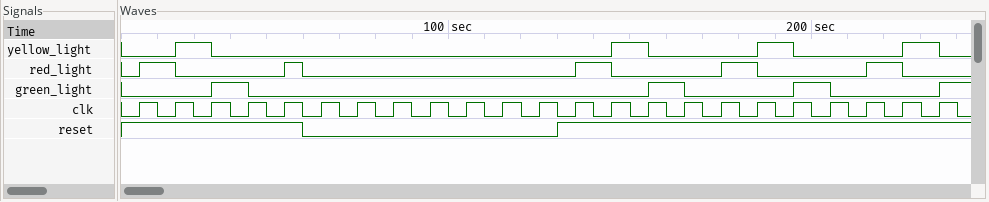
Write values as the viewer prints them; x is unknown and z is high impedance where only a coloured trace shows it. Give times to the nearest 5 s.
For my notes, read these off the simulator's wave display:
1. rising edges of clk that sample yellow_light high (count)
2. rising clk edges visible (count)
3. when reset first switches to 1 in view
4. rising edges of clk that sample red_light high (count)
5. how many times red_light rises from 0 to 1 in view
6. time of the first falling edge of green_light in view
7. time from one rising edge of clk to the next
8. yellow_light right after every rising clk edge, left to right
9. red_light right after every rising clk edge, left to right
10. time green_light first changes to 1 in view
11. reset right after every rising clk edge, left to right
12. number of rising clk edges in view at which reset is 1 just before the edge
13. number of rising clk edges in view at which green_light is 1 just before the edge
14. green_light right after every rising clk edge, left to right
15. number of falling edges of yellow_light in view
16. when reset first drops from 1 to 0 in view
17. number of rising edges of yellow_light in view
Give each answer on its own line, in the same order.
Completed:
4
23
130 s
4
5
45 s
10 s
0 1 0 0 0 0 0 0 0 0 0 0 0 1 0 0 0 1 0 0 0 1 0
1 0 0 0 1 0 0 0 0 0 0 0 1 0 0 0 1 0 0 0 1 0 0
35 s
1 1 1 1 1 0 0 0 0 0 0 0 1 1 1 1 1 1 1 1 1 1 1
16
3
0 0 1 0 0 0 0 0 0 0 0 0 0 0 1 0 0 0 1 0 0 0 1
4
60 s
4
